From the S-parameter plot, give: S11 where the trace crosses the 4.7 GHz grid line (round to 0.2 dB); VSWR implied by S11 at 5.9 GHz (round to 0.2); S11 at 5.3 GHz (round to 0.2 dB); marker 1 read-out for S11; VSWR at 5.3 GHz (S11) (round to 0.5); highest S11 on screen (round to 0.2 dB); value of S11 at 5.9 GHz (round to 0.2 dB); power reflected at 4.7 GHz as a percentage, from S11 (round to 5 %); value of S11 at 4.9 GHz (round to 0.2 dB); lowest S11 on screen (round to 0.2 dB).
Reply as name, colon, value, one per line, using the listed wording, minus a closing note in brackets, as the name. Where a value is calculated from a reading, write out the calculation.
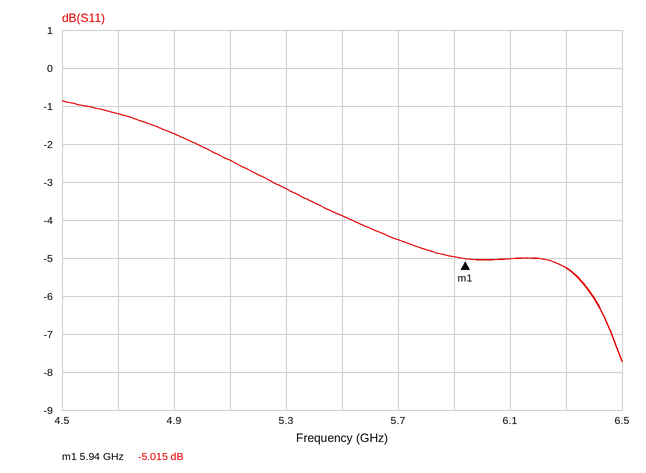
S11 where the trace crosses the 4.7 GHz grid line: -1.2 dB
VSWR implied by S11 at 5.9 GHz: |Γ| = 10^(-5/20) = 0.5623; VSWR = (1 + 0.5623)/(1 − 0.5623) ≈ 3.6
S11 at 5.3 GHz: -3.2 dB
marker 1 read-out for S11: -5.015 dB
VSWR at 5.3 GHz (S11): |Γ| = 10^(-3.2/20) = 0.6918; VSWR = (1 + 0.6918)/(1 − 0.6918) ≈ 5.5
highest S11 on screen: -0.8 dB
value of S11 at 5.9 GHz: -5.0 dB
power reflected at 4.7 GHz as a percentage, from S11: 10^(-1.2/10) ≈ 75.9 %, so 75 % to the nearest 5 %
value of S11 at 4.9 GHz: -1.8 dB
lowest S11 on screen: -7.8 dB
